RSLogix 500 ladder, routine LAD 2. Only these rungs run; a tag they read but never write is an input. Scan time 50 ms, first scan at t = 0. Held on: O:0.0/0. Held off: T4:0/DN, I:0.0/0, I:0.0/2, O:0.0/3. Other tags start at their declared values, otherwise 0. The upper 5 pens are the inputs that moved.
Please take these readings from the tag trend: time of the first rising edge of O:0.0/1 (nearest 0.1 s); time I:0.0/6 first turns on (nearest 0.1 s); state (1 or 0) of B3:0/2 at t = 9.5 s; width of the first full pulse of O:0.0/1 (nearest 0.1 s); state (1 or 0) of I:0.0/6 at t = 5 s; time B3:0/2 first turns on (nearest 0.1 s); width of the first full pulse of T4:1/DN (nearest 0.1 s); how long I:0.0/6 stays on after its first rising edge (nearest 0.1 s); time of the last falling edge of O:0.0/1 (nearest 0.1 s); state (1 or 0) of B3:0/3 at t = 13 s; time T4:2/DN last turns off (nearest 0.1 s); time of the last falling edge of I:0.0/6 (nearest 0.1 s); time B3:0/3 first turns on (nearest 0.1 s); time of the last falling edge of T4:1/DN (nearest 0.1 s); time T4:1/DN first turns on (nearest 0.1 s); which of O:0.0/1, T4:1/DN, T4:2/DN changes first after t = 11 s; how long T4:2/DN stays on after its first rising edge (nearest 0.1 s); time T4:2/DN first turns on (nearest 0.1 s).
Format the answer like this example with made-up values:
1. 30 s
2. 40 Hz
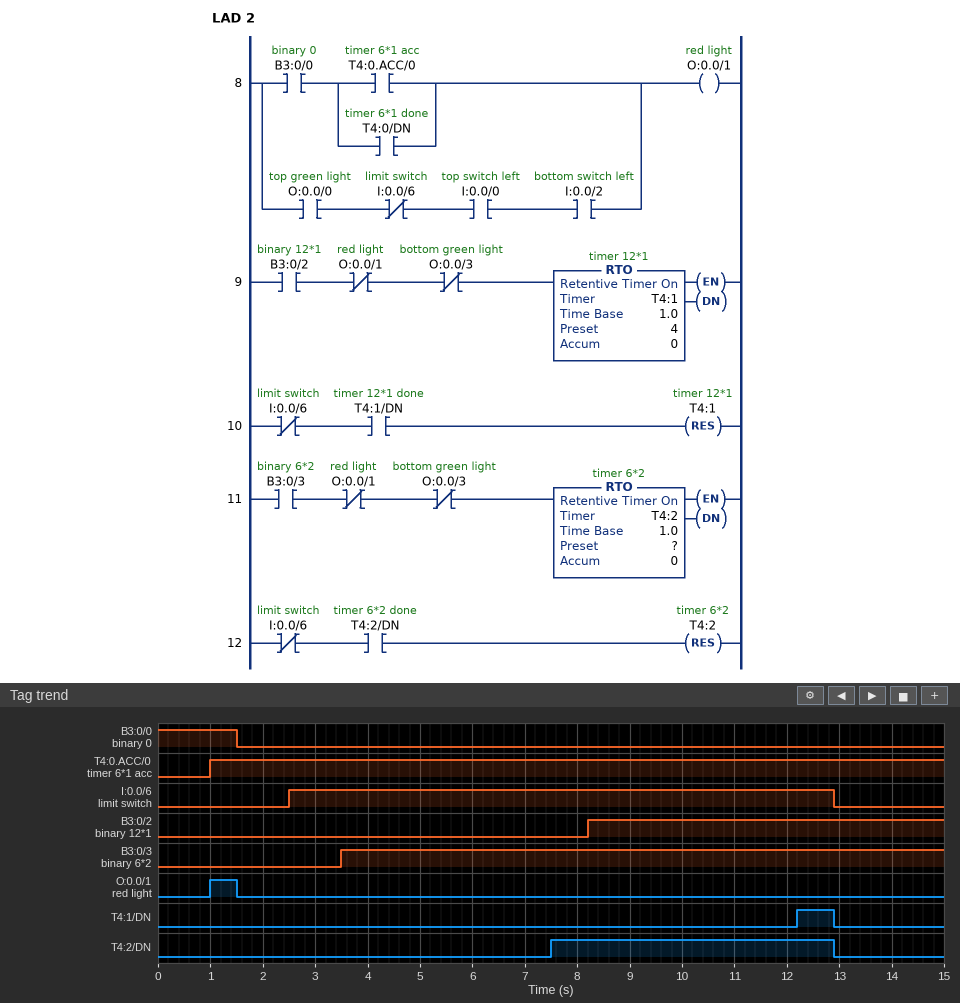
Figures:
1. 1.0 s
2. 2.5 s
3. 1
4. 0.5 s
5. 1
6. 8.2 s
7. 0.7 s
8. 10.4 s
9. 1.5 s
10. 1
11. 12.9 s
12. 12.9 s
13. 3.5 s
14. 12.9 s
15. 12.2 s
16. T4:1/DN
17. 5.4 s
18. 7.5 s
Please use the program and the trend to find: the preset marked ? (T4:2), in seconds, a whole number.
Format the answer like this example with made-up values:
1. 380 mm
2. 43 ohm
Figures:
1. 4 s
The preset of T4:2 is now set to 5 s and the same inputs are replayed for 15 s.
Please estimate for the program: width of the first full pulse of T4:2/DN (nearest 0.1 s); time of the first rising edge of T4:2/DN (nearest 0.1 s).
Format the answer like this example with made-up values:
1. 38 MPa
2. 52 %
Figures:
1. 4.4 s
2. 8.5 s
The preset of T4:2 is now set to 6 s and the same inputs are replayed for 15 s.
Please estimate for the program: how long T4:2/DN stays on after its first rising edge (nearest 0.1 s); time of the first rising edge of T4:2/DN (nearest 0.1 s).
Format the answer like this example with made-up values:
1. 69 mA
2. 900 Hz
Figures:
1. 3.4 s
2. 9.5 s
